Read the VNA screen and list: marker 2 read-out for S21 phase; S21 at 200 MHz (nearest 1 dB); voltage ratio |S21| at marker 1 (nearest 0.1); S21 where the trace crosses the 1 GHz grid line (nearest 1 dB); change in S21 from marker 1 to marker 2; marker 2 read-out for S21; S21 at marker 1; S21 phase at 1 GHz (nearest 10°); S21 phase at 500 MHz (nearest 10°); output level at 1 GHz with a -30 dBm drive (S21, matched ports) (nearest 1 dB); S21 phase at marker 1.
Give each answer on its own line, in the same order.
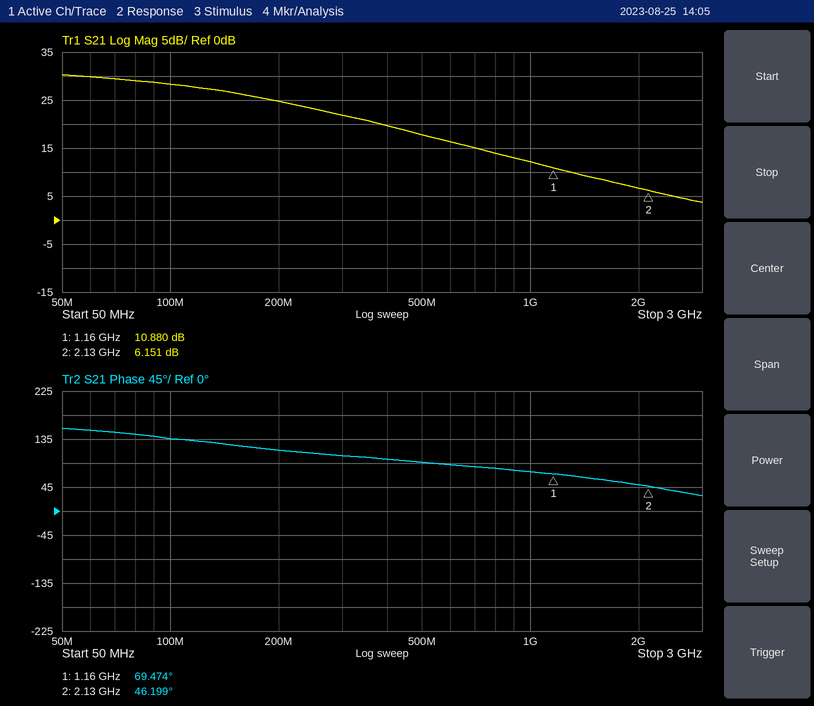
46.199°
25 dB
3.5
12 dB
-4.729 dB
6.151 dB
10.880 dB
70°
90°
-18 dBm
69.474°
